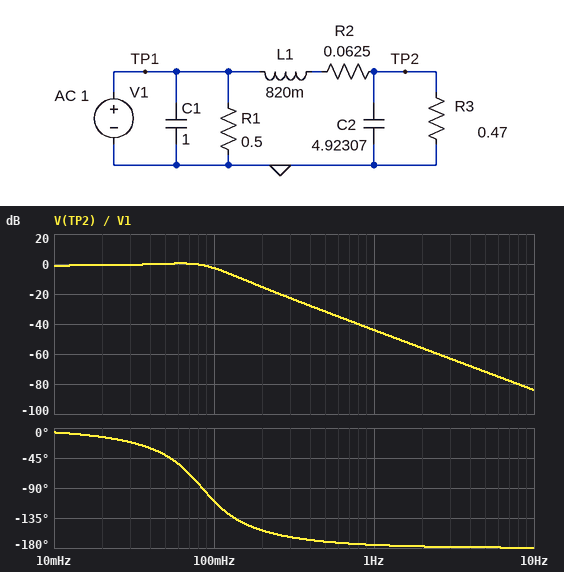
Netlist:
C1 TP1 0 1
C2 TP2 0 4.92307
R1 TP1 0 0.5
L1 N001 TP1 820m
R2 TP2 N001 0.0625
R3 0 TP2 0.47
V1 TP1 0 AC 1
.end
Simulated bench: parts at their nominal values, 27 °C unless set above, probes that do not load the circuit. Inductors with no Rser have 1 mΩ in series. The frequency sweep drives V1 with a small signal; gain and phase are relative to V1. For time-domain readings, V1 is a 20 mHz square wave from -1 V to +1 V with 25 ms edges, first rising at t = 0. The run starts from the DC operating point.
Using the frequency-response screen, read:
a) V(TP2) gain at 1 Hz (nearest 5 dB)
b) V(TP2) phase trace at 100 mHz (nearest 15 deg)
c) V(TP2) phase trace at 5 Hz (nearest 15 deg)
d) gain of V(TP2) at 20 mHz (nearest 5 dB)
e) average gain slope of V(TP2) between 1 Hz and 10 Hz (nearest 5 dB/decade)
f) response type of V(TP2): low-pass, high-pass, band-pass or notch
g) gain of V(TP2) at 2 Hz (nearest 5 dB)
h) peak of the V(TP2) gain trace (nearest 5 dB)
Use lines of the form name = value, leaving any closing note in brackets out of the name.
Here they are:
V(TP2) gain at 1 Hz = -45 dB
V(TP2) phase trace at 100 mHz = -105 deg
V(TP2) phase trace at 5 Hz = -180 deg
gain of V(TP2) at 20 mHz = 0 dB
average gain slope of V(TP2) between 1 Hz and 10 Hz = -40 dB/decade
response type of V(TP2): low-pass, high-pass, band-pass or notch = low-pass
gain of V(TP2) at 2 Hz = -55 dB
peak of the V(TP2) gain trace = 0 dB
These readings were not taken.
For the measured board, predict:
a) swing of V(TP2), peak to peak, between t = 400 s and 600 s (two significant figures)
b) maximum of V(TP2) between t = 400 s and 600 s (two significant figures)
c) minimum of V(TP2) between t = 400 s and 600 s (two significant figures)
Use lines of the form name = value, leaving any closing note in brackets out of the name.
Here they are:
swing of V(TP2), peak to peak, between t = 400 s and 600 s = 2.4 V
maximum of V(TP2) between t = 400 s and 600 s = 1.2 V
minimum of V(TP2) between t = 400 s and 600 s = -1.2 V
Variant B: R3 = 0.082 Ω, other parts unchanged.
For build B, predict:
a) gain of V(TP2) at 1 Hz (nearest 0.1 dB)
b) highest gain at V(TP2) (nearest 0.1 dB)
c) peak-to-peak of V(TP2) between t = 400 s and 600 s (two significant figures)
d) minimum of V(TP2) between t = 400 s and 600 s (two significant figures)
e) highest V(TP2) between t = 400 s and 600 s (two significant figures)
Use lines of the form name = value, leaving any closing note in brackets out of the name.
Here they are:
gain of V(TP2) at 1 Hz = -44.6 dB
highest gain at V(TP2) = -5.0 dB
peak-to-peak of V(TP2) between t = 400 s and 600 s = 1.1 V
minimum of V(TP2) between t = 400 s and 600 s = -550 mV
highest V(TP2) between t = 400 s and 600 s = 550 mV
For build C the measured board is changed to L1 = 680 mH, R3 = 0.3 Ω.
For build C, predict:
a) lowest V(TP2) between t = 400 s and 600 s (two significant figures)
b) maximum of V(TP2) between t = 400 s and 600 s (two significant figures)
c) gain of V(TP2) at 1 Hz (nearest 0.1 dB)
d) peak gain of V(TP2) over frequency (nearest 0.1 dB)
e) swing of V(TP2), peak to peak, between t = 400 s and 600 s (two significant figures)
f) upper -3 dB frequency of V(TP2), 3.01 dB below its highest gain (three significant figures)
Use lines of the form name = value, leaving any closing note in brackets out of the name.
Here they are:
lowest V(TP2) between t = 400 s and 600 s = -950 mV
maximum of V(TP2) between t = 400 s and 600 s = 950 mV
gain of V(TP2) at 1 Hz = -42.4 dB
peak gain of V(TP2) over frequency = -1.5 dB
swing of V(TP2), peak to peak, between t = 400 s and 600 s = 1.9 V
upper -3 dB frequency of V(TP2), 3.01 dB below its highest gain = 103 mHz
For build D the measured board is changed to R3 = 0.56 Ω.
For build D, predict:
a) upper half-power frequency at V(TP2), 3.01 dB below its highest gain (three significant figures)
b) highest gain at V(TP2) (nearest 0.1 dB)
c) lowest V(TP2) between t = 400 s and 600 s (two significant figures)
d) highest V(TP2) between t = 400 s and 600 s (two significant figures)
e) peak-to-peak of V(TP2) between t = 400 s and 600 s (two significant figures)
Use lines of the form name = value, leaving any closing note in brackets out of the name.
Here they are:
upper half-power frequency at V(TP2), 3.01 dB below its highest gain = 99.2 mHz
highest gain at V(TP2) = 1.4 dB
lowest V(TP2) between t = 400 s and 600 s = -1.3 V
highest V(TP2) between t = 400 s and 600 s = 1.3 V
peak-to-peak of V(TP2) between t = 400 s and 600 s = 2.6 V
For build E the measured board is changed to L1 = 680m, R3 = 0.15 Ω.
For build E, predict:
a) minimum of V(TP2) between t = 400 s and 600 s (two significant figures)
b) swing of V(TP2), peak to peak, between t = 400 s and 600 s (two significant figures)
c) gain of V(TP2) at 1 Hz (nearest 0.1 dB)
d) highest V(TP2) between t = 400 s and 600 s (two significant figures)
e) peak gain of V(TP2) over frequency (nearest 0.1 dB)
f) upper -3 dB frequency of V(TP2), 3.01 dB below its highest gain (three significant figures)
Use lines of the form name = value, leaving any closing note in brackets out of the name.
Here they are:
minimum of V(TP2) between t = 400 s and 600 s = -700 mV
swing of V(TP2), peak to peak, between t = 400 s and 600 s = 1.4 V
gain of V(TP2) at 1 Hz = -42.6 dB
highest V(TP2) between t = 400 s and 600 s = 700 mV
peak gain of V(TP2) over frequency = -3.1 dB
upper -3 dB frequency of V(TP2), 3.01 dB below its highest gain = 57.7 mHz
